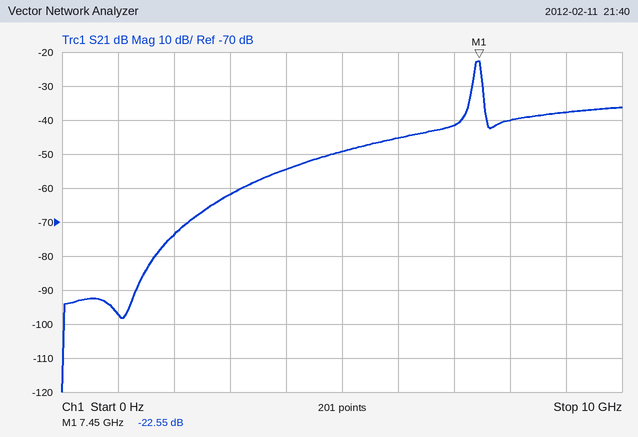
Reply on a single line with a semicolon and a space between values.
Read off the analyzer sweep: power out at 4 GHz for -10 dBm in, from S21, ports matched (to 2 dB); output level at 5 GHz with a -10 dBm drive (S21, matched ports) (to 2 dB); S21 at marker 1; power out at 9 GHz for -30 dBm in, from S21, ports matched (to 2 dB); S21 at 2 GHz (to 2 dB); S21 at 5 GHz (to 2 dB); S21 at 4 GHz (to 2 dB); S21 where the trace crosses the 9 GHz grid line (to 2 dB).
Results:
-64 dBm; -60 dBm; -22.55 dB; -68 dBm; -74 dB; -50 dB; -54 dB; -38 dB
